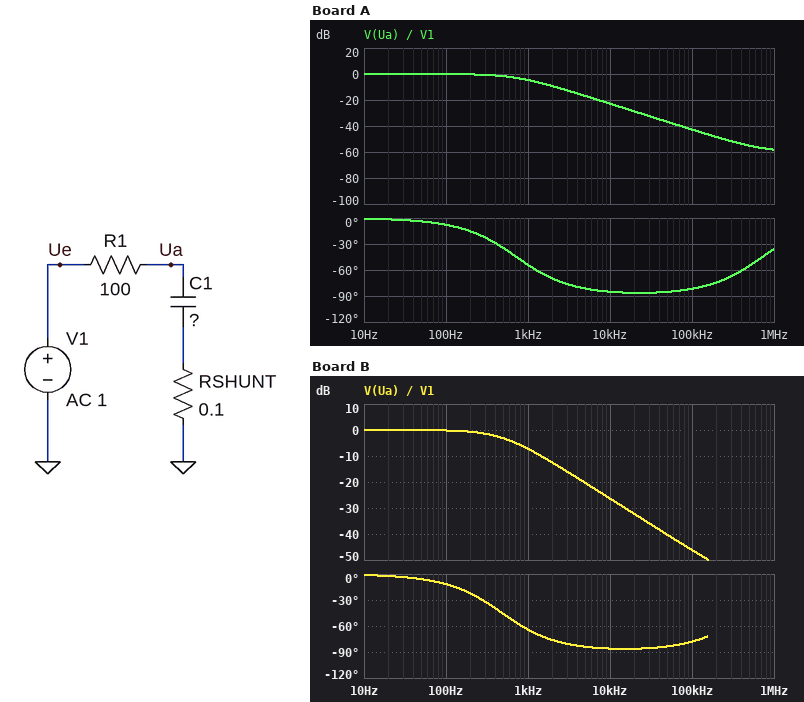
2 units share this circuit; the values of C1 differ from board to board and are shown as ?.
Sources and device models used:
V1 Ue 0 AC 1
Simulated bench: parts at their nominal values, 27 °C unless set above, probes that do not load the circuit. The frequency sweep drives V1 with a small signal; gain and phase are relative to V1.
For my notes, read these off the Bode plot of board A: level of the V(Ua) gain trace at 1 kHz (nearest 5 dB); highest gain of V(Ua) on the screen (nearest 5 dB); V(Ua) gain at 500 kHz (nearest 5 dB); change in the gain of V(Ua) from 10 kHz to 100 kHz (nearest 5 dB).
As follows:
-5 dB
0 dB
-55 dB
-20 dB
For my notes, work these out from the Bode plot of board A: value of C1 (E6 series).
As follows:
2.2 µF
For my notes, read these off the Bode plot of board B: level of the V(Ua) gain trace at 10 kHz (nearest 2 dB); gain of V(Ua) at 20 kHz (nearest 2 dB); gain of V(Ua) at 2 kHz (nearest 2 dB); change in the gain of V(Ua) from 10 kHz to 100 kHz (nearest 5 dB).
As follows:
-26 dB
-32 dB
-12 dB
-20 dB
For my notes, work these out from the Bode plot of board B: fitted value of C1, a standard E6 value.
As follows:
3.3 µF
